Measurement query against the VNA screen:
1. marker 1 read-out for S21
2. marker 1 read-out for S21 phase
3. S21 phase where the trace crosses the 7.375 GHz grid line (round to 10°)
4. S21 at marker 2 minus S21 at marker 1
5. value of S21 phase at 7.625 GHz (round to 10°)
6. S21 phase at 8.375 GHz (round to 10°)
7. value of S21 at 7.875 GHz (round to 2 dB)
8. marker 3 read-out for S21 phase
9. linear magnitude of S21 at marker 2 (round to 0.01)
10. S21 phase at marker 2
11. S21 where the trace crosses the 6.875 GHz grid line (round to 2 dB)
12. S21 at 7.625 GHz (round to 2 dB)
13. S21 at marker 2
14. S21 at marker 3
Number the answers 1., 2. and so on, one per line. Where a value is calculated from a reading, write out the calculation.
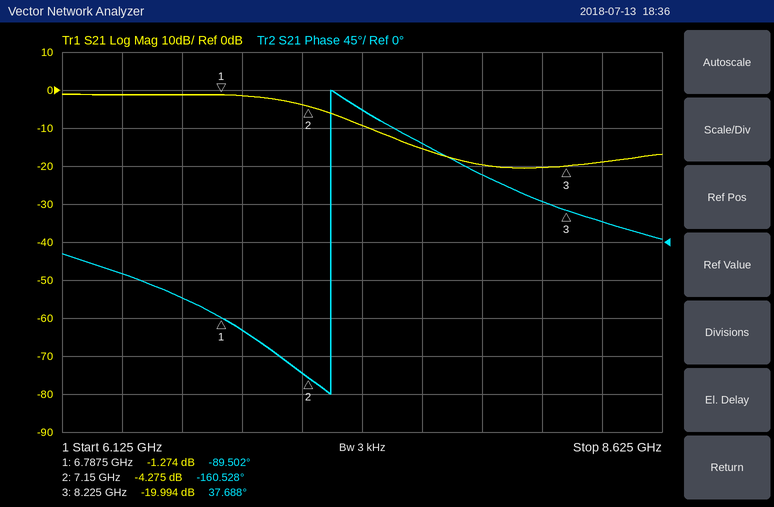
1. -1.274 dB
2. -89.502°
3. 160°
4. -4.275 − (-1.274) = -3.001 dB
5. 120°
6. 20°
7. -20 dB
8. 37.688°
9. 10^(-4.275/20) ≈ 0.61
10. -160.528°
11. -2 dB
12. -16 dB
13. -4.275 dB
14. -19.994 dB
